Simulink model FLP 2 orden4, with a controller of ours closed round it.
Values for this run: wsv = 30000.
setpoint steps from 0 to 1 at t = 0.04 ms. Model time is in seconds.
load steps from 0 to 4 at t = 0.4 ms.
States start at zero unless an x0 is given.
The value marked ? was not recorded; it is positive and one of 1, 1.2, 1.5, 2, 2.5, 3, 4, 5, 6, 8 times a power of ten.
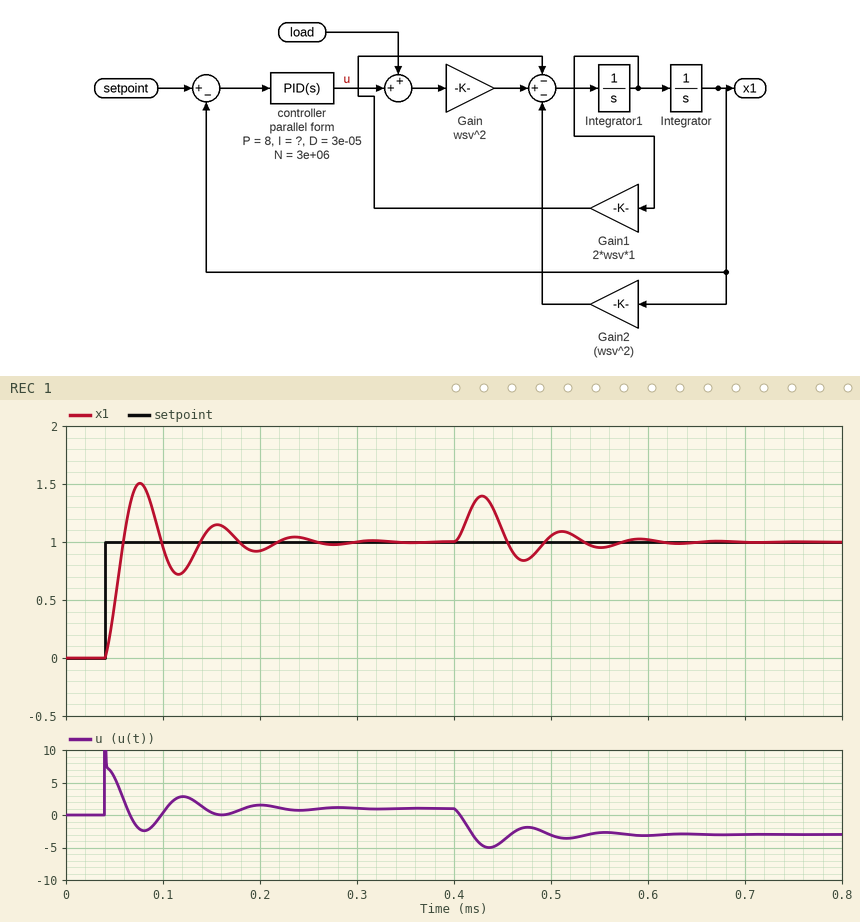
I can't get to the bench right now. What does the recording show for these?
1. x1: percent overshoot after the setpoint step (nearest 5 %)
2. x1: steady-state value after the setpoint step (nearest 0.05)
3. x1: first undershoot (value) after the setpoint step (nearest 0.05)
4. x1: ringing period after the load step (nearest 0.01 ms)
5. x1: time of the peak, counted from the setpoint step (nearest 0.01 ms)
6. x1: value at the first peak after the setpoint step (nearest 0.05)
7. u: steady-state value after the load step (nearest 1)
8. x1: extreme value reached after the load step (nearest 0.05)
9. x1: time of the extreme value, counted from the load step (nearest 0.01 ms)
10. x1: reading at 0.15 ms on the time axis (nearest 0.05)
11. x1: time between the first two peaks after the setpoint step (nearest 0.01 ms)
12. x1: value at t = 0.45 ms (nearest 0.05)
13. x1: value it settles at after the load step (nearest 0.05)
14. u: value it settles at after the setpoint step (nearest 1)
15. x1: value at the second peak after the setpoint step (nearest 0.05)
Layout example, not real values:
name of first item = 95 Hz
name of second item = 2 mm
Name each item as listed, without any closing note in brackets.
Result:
x1: percent overshoot after the setpoint step = 50 %
x1: steady-state value after the setpoint step = 1.00
x1: first undershoot (value) after the setpoint step = 0.70
x1: ringing period after the load step = 0.08 ms
x1: time of the peak, counted from the setpoint step = 0.04 ms
x1: value at the first peak after the setpoint step = 1.50
u: steady-state value after the load step = -3
x1: extreme value reached after the load step = 1.40
x1: time of the extreme value, counted from the load step = 0.03 ms
x1: reading at 0.15 ms on the time axis = 1.15
x1: time between the first two peaks after the setpoint step = 0.08 ms
x1: value at t = 0.45 ms = 1.10
x1: value it settles at after the load step = 1.00
u: value it settles at after the setpoint step = 1
x1: value at the second peak after the setpoint step = 1.15
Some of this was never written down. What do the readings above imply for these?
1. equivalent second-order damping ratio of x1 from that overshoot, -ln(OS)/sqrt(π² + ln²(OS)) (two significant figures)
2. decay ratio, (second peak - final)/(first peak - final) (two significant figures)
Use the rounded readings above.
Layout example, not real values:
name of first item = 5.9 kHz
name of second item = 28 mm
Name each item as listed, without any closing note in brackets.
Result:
equivalent second-order damping ratio of x1 from that overshoot, -ln(OS)/sqrt(π² + ln²(OS)) = 0.22
decay ratio, (second peak - final)/(first peak - final) = 0.30
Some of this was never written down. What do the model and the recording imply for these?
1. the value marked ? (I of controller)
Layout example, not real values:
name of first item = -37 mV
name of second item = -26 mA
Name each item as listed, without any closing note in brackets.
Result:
the value marked ? = 400000
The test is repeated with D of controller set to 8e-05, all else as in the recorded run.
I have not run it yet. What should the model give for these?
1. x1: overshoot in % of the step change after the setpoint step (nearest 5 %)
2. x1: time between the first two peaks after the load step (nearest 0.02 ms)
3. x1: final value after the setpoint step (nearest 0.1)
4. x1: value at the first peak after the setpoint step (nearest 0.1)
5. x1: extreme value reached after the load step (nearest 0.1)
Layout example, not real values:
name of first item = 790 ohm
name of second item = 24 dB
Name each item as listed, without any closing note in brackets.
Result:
x1: overshoot in % of the step change after the setpoint step = 25 %
x1: time between the first two peaks after the load step = 0.10 ms
x1: final value after the setpoint step = 1.0
x1: value at the first peak after the setpoint step = 1.3
x1: extreme value reached after the load step = 1.3
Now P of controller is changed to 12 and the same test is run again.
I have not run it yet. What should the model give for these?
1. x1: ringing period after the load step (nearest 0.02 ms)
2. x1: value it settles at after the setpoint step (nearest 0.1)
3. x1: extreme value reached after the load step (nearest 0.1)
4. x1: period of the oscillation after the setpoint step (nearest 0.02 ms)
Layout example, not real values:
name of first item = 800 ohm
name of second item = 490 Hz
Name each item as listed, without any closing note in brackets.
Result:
x1: ringing period after the load step = 0.06 ms
x1: value it settles at after the setpoint step = 1.0
x1: extreme value reached after the load step = 1.3
x1: period of the oscillation after the setpoint step = 0.06 ms
